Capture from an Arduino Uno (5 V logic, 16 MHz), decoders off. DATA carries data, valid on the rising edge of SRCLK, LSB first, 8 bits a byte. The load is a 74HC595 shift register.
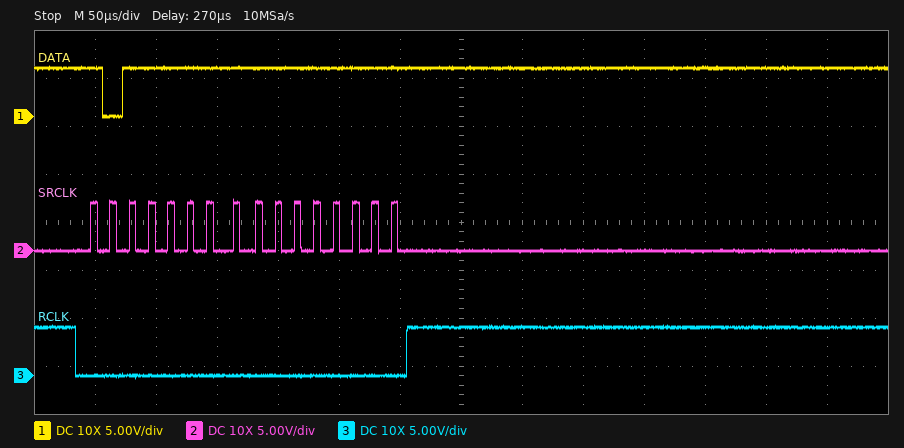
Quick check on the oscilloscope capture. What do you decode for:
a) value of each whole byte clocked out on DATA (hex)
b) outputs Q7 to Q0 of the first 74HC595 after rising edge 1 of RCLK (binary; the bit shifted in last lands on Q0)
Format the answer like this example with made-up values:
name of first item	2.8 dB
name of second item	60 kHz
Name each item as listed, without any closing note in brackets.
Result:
value of each whole byte clocked out on DATA	FD FF
outputs Q7 to Q0 of the first 74HC595 after rising edge 1 of RCLK	11111111
